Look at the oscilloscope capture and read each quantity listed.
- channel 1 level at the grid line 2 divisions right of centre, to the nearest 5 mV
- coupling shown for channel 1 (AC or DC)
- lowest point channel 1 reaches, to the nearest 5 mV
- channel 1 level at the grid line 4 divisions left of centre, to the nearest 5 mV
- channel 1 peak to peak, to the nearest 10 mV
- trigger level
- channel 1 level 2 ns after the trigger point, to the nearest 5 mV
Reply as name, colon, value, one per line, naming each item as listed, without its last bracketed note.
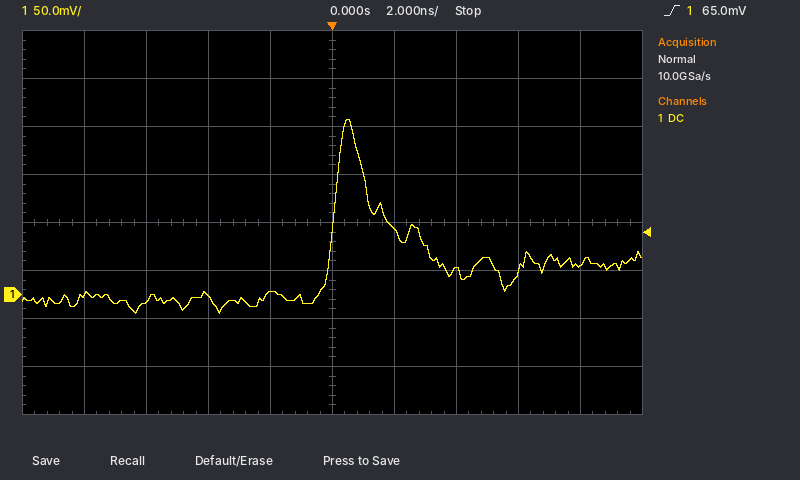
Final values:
channel 1 level at the grid line 2 divisions right of centre, to the nearest 5 mV: 25 mV
coupling shown for channel 1: DC
lowest point channel 1 reaches, to the nearest 5 mV: -20 mV
channel 1 level at the grid line 4 divisions left of centre, to the nearest 5 mV: 0 mV
channel 1 peak to peak, to the nearest 10 mV: 200 mV
trigger level: 65.0 mV
channel 1 level 2 ns after the trigger point, to the nearest 5 mV: 70 mV
